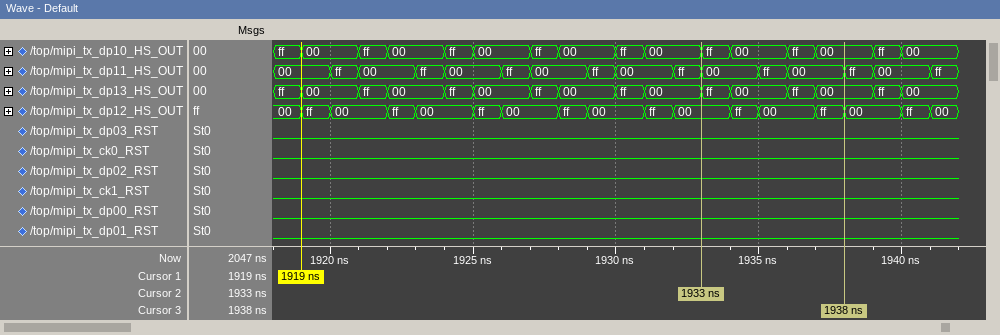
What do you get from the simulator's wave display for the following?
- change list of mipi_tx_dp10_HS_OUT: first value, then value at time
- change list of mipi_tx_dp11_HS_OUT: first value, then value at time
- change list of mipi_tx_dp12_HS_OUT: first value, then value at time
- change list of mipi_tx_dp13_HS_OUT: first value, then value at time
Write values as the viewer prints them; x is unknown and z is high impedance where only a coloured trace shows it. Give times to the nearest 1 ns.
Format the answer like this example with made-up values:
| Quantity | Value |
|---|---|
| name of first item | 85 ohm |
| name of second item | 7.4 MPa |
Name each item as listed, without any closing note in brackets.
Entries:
| Quantity | Value |
|---|---|
| change list of mipi_tx_dp10_HS_OUT: first value, then value at time | ff, 00 at 1919 ns, ff at 1921 ns, 00 at 1922 ns, ff at 1924 ns, 00 at 1925 ns, ff at 1927 ns, 00 at 1928 ns, ff at 1930 ns, 00 at 1931 ns, ff at 1933 ns, 00 at 1934 ns, ff at 1936 ns, 00 at 1937 ns, ff at 1939 ns, 00 at 1940 ns |
| change list of mipi_tx_dp11_HS_OUT: first value, then value at time | 00, ff at 1920 ns, 00 at 1921 ns, ff at 1923 ns, 00 at 1924 ns, ff at 1926 ns, 00 at 1927 ns, ff at 1929 ns, 00 at 1930 ns, ff at 1932 ns, 00 at 1933 ns, ff at 1935 ns, 00 at 1936 ns, ff at 1938 ns, 00 at 1939 ns, ff at 1941 ns |
| change list of mipi_tx_dp12_HS_OUT: first value, then value at time | 00, ff at 1919 ns, 00 at 1920 ns, ff at 1922 ns, 00 at 1923 ns, ff at 1925 ns, 00 at 1926 ns, ff at 1928 ns, 00 at 1929 ns, ff at 1931 ns, 00 at 1932 ns, ff at 1934 ns, 00 at 1935 ns, ff at 1937 ns, 00 at 1938 ns, ff at 1940 ns, 00 at 1941 ns |
| change list of mipi_tx_dp13_HS_OUT: first value, then value at time | ff, 00 at 1919 ns, ff at 1921 ns, 00 at 1922 ns, ff at 1924 ns, 00 at 1925 ns, ff at 1927 ns, 00 at 1928 ns, ff at 1930 ns, 00 at 1931 ns, ff at 1933 ns, 00 at 1934 ns, ff at 1936 ns, 00 at 1937 ns, ff at 1939 ns, 00 at 1940 ns |
